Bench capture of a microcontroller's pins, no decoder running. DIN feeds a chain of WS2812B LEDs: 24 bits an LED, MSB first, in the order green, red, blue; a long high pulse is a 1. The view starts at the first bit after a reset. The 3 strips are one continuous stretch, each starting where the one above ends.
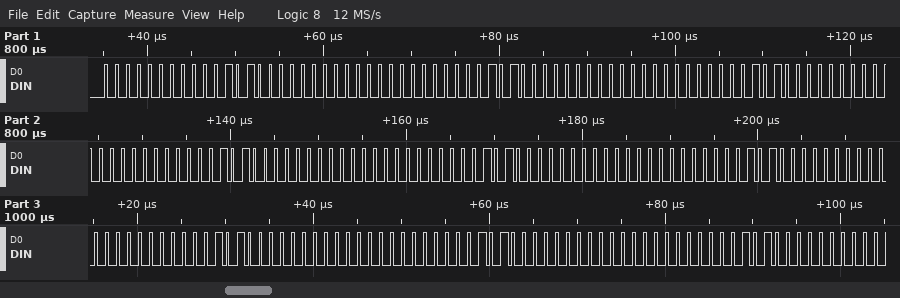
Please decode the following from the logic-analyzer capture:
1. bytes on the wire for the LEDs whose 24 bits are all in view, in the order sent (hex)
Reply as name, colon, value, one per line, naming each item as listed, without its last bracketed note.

bytes on the wire for the LEDs whose 24 bits are all in view, in the order sent: 00 14 00 00 14 00 00 14 00 00 14 00 00 14 00 00 14 00 00 14 00 00 14 00 00 14 00
